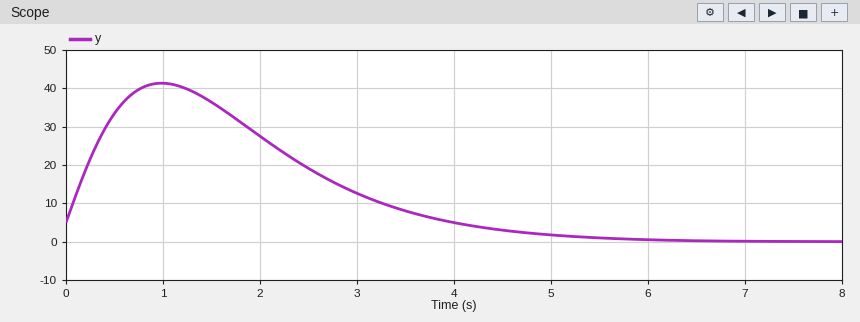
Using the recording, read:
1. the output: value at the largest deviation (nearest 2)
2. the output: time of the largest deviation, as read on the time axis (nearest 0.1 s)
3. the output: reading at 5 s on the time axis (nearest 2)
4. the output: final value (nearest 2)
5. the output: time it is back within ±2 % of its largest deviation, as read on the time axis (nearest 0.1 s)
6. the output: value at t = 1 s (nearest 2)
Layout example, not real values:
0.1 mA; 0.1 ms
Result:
42; 1.0 s; 2; 0; 5.7 s; 42
